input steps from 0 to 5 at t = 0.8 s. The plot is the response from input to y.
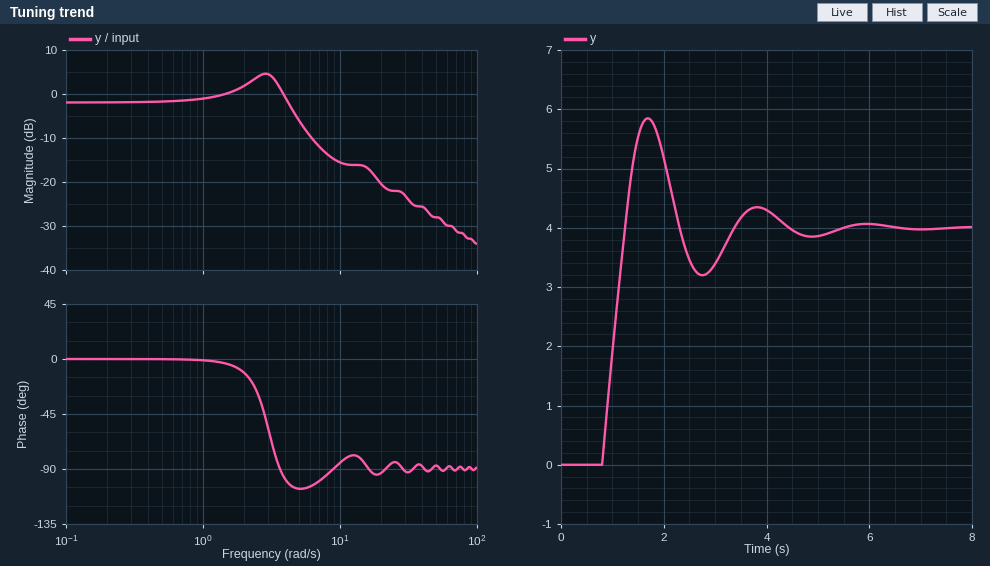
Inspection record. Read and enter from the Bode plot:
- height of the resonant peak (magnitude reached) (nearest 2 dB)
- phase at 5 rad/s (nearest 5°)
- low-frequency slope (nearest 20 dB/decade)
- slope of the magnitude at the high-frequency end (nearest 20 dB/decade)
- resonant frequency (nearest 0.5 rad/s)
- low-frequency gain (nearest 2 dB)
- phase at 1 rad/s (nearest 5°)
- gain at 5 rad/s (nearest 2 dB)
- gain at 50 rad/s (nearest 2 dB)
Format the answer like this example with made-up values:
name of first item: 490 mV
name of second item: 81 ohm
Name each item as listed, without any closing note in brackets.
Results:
height of the resonant peak (magnitude reached): 4 dB
phase at 5 rad/s: -105°
low-frequency slope: 0 dB/decade
slope of the magnitude at the high-frequency end: -20 dB/decade
resonant frequency: 3.0 rad/s
low-frequency gain: -2 dB
phase at 1 rad/s: 0°
gain at 5 rad/s: -6 dB
gain at 50 rad/s: -28 dB
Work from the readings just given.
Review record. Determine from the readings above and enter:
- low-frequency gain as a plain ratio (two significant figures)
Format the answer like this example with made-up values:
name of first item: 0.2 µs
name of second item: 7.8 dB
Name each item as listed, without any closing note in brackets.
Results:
low-frequency gain as a plain ratio: 0.79
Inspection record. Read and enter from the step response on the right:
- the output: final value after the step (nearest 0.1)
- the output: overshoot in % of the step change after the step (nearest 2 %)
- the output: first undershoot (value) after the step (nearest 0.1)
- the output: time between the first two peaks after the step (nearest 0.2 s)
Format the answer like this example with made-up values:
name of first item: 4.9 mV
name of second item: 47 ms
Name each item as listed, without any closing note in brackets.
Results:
the output: final value after the step: 4.0
the output: overshoot in % of the step change after the step: 46 %
the output: first undershoot (value) after the step: 3.2
the output: time between the first two peaks after the step: 2.2 s
